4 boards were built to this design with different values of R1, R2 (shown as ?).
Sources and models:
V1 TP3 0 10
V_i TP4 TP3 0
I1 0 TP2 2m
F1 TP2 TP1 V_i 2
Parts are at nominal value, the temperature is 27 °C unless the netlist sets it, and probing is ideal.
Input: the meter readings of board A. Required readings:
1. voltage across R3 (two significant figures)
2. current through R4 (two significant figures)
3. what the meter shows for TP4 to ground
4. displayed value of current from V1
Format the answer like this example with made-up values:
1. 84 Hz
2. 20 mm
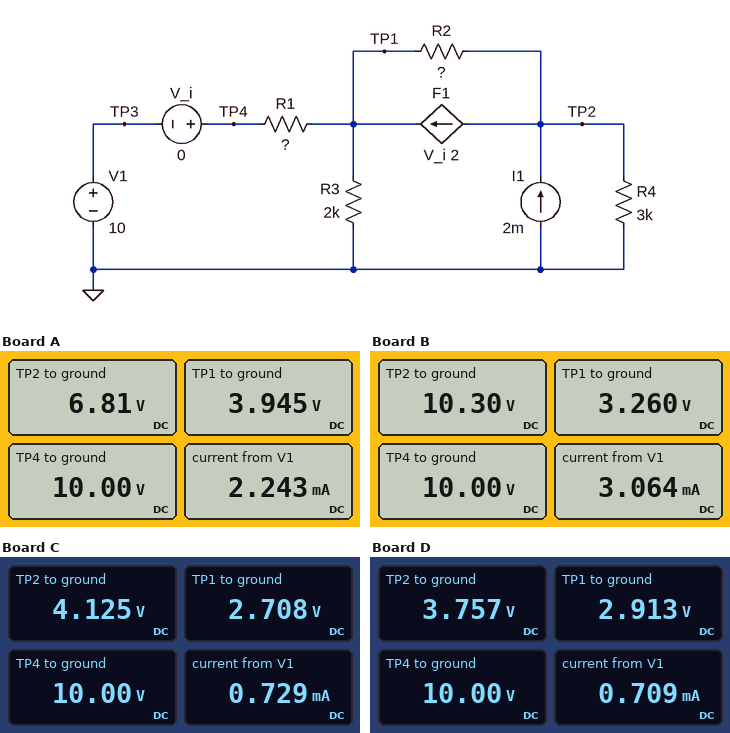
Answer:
1. 3.9 V
2. 2.3 mA
3. 10.00 V
4. 2.243 mA
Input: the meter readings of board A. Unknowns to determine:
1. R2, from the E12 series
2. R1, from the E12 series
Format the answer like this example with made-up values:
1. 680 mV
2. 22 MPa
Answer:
1. 680 Ω
2. 2.7 kΩ
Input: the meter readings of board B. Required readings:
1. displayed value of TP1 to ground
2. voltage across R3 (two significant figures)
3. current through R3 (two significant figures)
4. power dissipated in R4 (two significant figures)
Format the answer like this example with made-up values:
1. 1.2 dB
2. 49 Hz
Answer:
1. 3.260 V
2. 3.3 V
3. 1.6 mA
4. 35 mW
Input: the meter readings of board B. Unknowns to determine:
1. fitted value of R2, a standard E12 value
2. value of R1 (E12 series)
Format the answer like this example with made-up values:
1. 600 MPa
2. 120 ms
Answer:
1. 1.5 kΩ
2. 2.2 kΩ
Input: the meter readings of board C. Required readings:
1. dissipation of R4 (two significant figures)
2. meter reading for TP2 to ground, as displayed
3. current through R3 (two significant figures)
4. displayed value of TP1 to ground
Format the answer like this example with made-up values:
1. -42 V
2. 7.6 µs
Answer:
1. 5.7 mW
2. 4.125 V
3. 1.4 mA
4. 2.708 V
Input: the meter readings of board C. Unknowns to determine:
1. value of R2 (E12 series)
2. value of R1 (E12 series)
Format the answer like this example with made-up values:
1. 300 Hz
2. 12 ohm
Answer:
1. 680 Ω
2. 10 kΩ
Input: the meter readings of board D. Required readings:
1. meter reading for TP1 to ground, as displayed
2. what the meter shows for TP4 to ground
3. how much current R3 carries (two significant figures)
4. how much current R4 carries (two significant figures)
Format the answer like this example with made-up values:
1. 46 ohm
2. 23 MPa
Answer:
1. 2.913 V
2. 10.00 V
3. 1.5 mA
4. 1.3 mA
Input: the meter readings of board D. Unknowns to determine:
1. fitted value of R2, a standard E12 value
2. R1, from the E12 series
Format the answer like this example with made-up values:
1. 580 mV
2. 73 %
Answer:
1. 390 Ω
2. 10 kΩ
